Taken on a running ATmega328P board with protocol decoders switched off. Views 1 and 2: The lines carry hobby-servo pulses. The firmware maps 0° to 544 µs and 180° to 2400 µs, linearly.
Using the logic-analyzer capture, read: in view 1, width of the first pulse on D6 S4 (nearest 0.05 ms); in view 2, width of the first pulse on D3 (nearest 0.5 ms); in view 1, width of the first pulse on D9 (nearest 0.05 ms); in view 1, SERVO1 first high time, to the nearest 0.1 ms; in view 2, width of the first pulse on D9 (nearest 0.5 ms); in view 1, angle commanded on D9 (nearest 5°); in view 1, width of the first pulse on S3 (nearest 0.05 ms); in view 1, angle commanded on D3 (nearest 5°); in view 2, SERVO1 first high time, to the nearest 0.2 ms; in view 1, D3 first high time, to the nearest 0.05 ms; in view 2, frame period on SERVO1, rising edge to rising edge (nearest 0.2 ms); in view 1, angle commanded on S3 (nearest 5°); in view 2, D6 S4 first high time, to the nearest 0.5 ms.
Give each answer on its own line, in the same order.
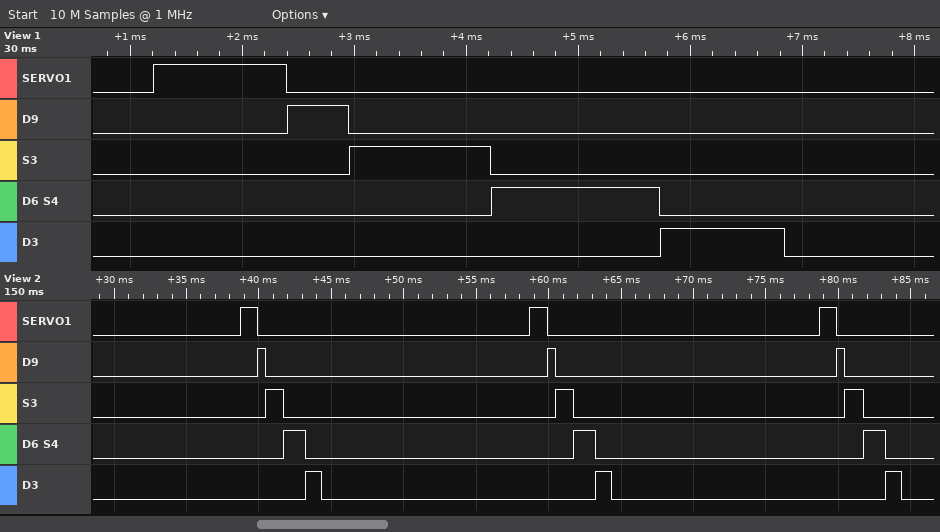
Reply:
1.50 ms
1.0 ms
0.55 ms
1.2 ms
0.5 ms
0°
1.25 ms
55°
1.2 ms
1.10 ms
20.0 ms
70°
1.5 ms
